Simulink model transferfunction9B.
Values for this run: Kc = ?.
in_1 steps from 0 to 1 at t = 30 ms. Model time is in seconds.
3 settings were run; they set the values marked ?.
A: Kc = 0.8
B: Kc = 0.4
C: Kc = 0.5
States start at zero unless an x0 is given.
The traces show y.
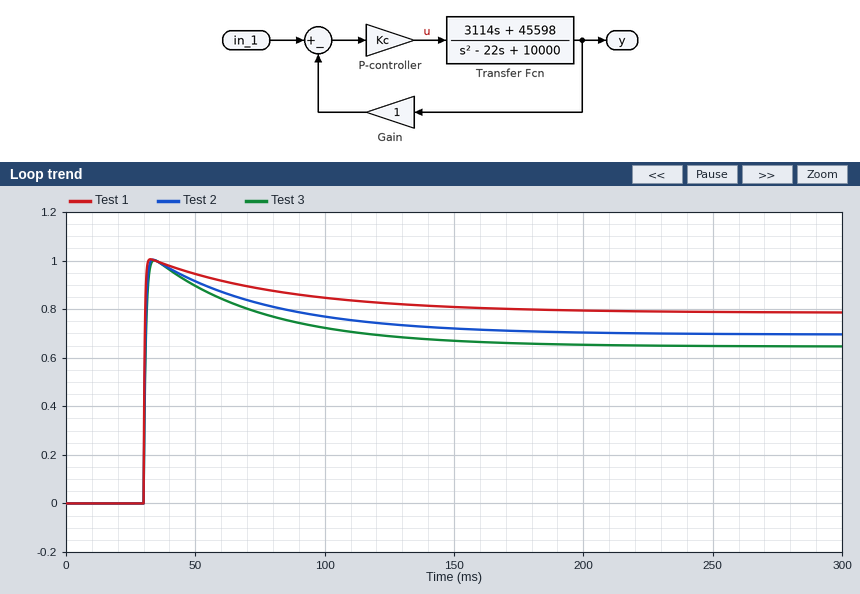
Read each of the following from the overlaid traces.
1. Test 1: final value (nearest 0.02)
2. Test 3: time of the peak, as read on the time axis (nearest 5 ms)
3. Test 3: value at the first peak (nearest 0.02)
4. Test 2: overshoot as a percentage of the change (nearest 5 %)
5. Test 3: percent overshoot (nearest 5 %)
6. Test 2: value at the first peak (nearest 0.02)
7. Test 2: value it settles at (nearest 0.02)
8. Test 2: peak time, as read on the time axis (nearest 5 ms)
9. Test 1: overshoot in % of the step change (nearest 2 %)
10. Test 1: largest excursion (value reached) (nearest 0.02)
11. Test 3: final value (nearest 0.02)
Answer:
0.78
35 ms
1.00
45 %
55 %
1.00
0.70
35 ms
28 %
1.00
0.64
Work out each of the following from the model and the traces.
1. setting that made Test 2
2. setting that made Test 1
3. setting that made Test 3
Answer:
C
A
B
